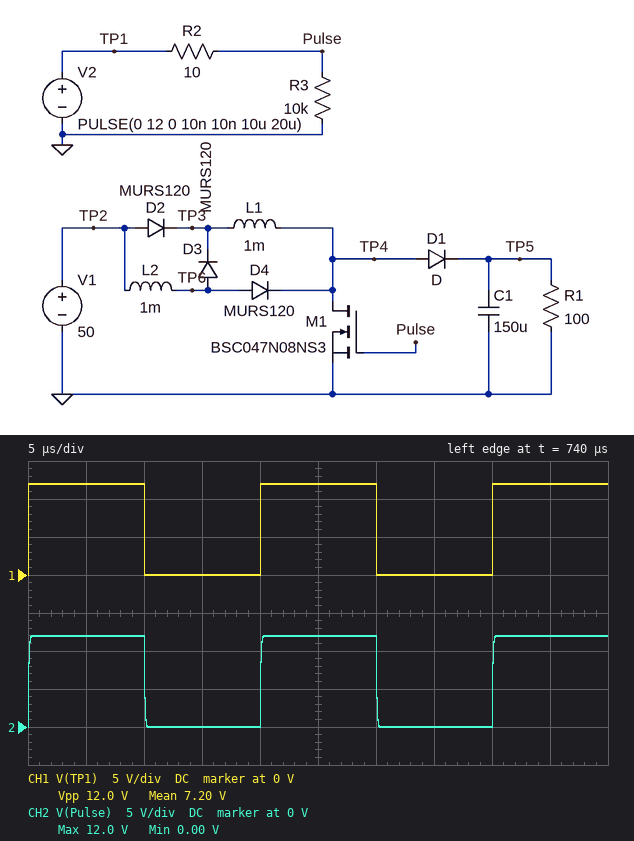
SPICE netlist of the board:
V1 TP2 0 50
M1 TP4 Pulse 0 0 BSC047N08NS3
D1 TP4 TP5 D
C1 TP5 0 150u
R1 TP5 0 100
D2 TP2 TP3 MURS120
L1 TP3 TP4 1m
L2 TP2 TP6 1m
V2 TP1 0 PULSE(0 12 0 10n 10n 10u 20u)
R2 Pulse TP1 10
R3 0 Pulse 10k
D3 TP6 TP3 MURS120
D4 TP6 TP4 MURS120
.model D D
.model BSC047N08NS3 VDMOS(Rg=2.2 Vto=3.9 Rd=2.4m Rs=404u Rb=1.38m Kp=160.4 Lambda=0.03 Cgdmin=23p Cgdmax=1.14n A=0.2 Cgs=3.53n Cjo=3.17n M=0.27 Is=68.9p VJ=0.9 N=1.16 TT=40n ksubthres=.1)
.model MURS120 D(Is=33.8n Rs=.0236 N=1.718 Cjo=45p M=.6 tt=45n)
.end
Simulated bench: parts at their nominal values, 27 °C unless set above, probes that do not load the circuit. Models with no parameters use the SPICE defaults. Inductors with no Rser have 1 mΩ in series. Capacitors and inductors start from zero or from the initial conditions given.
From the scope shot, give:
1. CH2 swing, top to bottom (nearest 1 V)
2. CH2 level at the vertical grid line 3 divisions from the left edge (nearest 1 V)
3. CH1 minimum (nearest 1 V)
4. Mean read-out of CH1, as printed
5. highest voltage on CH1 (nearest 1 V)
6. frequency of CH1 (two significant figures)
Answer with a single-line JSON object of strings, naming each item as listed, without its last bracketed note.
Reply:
{"CH2 swing, top to bottom": "12 V", "CH2 level at the vertical grid line 3 divisions from the left edge": "0 V", "CH1 minimum": "0 V", "Mean read-out of CH1, as printed": "7.20 V", "highest voltage on CH1": "12 V", "frequency of CH1": "50 kHz"}
